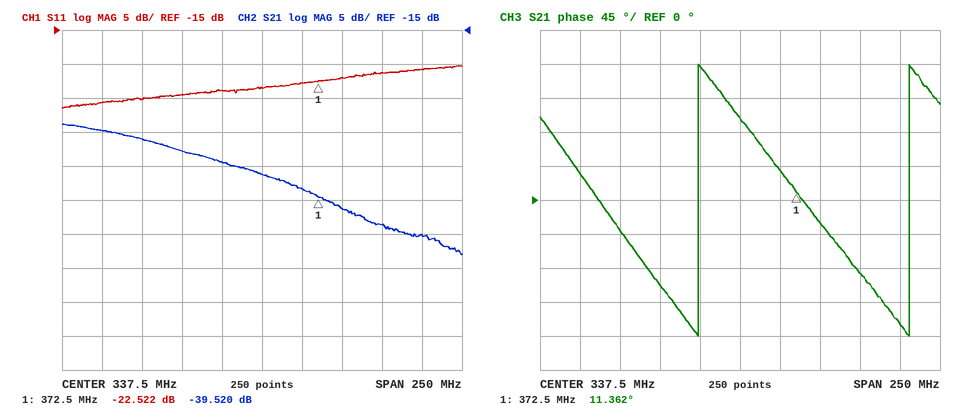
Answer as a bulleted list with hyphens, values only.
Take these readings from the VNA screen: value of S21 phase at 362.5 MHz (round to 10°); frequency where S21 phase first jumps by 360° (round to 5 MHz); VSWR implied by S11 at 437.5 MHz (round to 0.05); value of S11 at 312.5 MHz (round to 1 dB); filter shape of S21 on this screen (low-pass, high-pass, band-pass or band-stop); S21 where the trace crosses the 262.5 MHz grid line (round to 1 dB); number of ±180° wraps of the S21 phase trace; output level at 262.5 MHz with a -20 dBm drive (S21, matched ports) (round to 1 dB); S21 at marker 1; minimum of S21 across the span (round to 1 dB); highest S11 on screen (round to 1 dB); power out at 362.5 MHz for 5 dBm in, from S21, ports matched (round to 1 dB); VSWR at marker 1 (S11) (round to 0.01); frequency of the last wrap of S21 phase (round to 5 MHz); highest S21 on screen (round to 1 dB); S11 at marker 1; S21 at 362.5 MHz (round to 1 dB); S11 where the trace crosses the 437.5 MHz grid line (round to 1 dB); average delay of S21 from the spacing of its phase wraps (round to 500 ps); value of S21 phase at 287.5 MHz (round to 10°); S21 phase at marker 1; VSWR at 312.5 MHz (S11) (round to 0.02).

- 40°
- 310 MHz
- 1.20
- -24 dB
- low-pass
- -31 dB
- 2
- -51 dBm
- -39.520 dB
- -48 dB
- -20 dB
- -33 dBm
- 1.16
- 445 MHz
- -29 dB
- -22.522 dB
- -38 dB
- -21 dB
- 7.5 ns
- -110°
- 11.362°
- 1.14
